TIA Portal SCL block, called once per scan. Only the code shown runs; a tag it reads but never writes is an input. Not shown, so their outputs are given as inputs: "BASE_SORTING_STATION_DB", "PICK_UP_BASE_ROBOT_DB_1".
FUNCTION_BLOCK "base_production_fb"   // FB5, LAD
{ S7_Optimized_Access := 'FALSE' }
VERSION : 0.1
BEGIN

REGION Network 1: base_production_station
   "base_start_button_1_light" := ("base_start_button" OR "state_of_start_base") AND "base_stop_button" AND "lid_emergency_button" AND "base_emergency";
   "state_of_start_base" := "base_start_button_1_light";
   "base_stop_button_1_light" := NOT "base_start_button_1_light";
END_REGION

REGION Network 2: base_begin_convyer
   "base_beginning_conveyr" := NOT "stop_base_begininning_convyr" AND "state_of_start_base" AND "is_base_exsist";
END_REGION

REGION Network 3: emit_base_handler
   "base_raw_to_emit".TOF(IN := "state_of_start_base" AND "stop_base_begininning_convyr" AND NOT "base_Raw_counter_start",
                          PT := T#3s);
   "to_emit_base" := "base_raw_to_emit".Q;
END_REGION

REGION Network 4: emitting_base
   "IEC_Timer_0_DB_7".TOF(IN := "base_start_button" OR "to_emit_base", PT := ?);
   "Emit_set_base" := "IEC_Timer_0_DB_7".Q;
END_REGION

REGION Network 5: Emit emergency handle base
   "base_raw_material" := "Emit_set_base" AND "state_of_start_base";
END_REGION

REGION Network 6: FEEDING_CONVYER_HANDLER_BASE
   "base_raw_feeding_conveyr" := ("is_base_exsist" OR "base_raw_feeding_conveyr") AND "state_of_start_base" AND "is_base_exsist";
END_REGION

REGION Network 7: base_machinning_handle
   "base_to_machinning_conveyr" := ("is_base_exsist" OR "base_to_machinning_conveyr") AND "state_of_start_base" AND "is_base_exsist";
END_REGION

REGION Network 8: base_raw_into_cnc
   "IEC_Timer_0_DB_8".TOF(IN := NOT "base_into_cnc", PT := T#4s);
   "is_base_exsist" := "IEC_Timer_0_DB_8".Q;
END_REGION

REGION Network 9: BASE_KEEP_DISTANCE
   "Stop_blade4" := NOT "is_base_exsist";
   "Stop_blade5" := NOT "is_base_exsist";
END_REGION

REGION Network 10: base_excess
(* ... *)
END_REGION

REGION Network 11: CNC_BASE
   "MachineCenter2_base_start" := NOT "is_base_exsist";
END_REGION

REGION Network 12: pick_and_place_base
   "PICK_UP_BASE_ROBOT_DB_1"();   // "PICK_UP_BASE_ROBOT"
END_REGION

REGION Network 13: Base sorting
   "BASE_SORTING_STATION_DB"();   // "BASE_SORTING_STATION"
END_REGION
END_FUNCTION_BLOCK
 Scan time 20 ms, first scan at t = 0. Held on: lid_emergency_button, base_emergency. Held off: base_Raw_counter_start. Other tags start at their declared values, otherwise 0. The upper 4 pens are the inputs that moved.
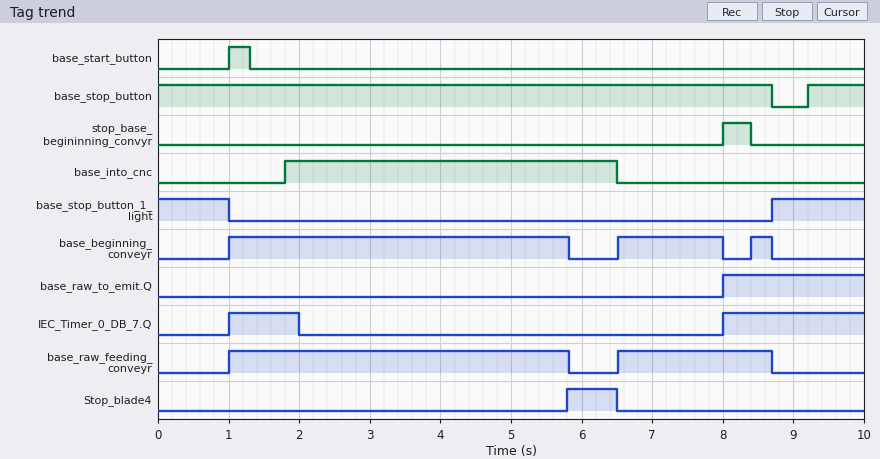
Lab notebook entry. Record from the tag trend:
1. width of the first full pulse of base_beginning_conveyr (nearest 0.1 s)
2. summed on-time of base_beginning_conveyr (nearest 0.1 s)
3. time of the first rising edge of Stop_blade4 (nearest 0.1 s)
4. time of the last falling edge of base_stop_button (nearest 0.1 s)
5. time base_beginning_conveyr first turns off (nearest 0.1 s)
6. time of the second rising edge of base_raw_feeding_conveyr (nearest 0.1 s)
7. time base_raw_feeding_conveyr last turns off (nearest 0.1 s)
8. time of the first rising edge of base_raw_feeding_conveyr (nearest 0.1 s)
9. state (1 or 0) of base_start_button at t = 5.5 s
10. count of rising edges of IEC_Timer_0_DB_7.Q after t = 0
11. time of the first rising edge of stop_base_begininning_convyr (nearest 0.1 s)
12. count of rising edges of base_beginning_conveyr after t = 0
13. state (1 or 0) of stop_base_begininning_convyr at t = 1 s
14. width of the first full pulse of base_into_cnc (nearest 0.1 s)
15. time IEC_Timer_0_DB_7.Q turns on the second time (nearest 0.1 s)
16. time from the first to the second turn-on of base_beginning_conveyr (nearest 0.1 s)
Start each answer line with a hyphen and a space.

- 4.8 s
- 6.6 s
- 5.8 s
- 8.7 s
- 5.8 s
- 6.5 s
- 8.7 s
- 1.0 s
- 0
- 2
- 8.0 s
- 3
- 0
- 4.7 s
- 8.0 s
- 5.5 s
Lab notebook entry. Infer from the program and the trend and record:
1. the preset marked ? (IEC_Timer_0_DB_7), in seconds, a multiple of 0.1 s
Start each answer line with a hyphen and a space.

- 0.7 s
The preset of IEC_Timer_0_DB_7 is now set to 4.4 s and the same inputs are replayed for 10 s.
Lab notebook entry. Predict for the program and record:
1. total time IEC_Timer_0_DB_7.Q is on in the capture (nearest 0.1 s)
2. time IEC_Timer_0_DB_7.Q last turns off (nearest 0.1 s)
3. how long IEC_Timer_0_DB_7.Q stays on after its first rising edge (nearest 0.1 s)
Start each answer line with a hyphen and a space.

- 6.7 s
- 5.7 s
- 4.7 s
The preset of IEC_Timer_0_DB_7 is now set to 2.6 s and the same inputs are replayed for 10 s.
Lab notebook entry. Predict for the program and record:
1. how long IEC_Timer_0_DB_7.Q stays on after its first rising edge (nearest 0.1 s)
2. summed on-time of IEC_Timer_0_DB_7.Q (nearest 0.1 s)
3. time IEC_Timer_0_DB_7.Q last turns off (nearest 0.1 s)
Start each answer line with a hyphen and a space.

- 2.9 s
- 4.9 s
- 3.9 s
